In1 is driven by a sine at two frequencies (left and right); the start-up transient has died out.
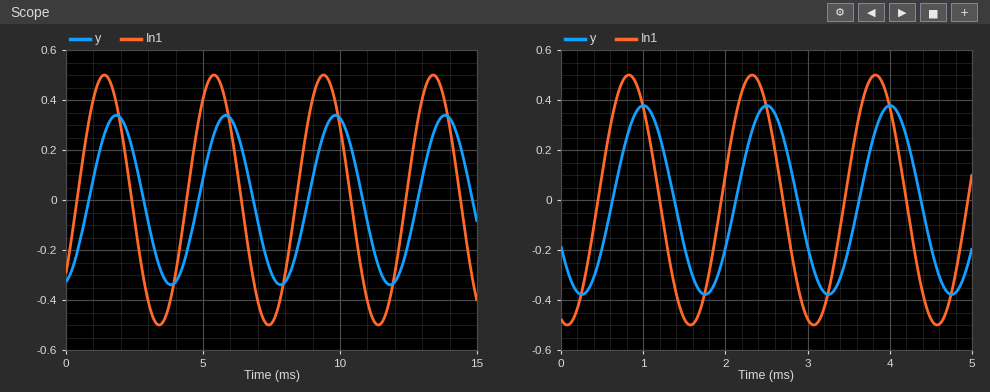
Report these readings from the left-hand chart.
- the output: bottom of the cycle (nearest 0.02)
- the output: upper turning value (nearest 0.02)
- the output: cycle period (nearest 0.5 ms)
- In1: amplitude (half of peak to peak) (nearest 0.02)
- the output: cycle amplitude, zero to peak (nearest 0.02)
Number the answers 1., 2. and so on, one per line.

1. -0.34
2. 0.34
3. 4.0 ms
4. 0.50
5. 0.34
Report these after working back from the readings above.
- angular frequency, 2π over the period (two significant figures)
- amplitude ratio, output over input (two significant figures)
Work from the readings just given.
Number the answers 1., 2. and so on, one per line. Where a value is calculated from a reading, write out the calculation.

1. 2π / 4 = 1.6 rad/ms
2. 0.34 / 0.5 = 0.68
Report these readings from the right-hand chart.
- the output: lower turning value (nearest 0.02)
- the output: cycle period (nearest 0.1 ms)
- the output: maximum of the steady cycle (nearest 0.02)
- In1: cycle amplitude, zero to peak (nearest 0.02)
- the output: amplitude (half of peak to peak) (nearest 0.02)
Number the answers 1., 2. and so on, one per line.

1. -0.38
2. 1.5 ms
3. 0.38
4. 0.50
5. 0.38
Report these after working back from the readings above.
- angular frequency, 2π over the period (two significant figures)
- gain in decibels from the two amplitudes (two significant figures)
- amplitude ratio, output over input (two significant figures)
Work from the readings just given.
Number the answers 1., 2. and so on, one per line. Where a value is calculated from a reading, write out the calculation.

1. 2π / 1.5 = 4.2 rad/ms
2. 20 log10(0.38 / 0.5) = -2.4 dB
3. 0.38 / 0.5 = 0.76
